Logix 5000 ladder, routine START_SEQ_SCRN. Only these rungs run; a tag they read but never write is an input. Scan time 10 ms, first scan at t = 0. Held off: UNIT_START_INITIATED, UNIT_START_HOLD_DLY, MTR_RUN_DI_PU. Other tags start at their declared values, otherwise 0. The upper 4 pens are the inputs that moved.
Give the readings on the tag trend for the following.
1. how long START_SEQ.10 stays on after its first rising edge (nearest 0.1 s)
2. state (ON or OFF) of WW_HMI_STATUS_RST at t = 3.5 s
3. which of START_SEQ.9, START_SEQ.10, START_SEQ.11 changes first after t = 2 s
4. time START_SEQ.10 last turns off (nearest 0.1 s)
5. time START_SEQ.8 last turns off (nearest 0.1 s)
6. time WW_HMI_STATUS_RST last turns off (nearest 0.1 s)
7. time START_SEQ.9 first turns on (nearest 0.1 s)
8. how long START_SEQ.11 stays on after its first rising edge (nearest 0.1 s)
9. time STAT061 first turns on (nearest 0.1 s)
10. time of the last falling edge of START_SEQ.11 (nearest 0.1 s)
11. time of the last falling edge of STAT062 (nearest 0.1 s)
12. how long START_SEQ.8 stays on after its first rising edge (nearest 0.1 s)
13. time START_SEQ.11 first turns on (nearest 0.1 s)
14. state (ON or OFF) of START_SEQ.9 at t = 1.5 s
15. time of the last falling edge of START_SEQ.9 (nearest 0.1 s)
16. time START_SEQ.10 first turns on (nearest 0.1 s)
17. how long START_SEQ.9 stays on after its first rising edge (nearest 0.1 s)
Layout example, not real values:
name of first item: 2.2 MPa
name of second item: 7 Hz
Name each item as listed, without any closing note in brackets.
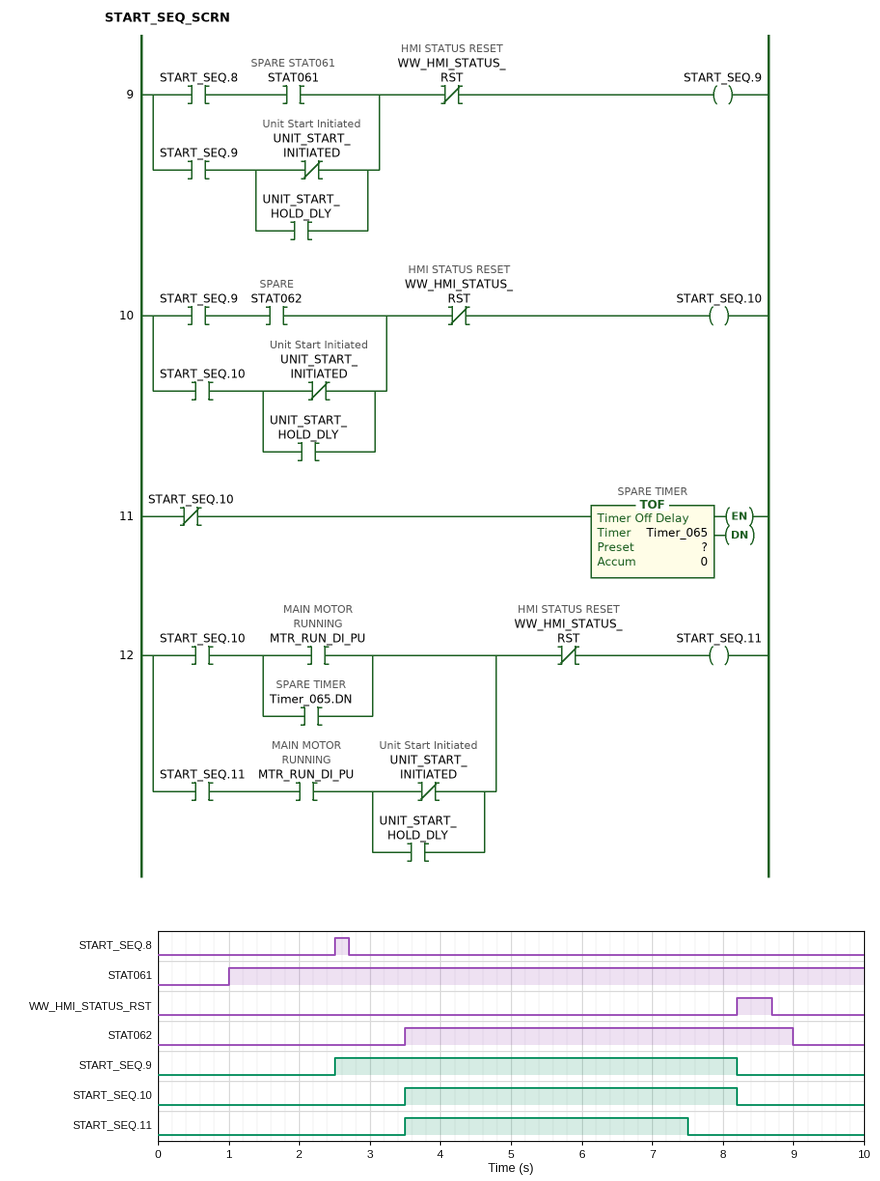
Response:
how long START_SEQ.10 stays on after its first rising edge: 4.7 s
state (ON or OFF) of WW_HMI_STATUS_RST at t = 3.5 s: OFF
which of START_SEQ.9, START_SEQ.10, START_SEQ.11 changes first after t = 2 s: START_SEQ.9
time START_SEQ.10 last turns off: 8.2 s
time START_SEQ.8 last turns off: 2.7 s
time WW_HMI_STATUS_RST last turns off: 8.7 s
time START_SEQ.9 first turns on: 2.5 s
how long START_SEQ.11 stays on after its first rising edge: 4.0 s
time STAT061 first turns on: 1.0 s
time of the last falling edge of START_SEQ.11: 7.5 s
time of the last falling edge of STAT062: 9.0 s
how long START_SEQ.8 stays on after its first rising edge: 0.2 s
time START_SEQ.11 first turns on: 3.5 s
state (ON or OFF) of START_SEQ.9 at t = 1.5 s: OFF
time of the last falling edge of START_SEQ.9: 8.2 s
time START_SEQ.10 first turns on: 3.5 s
how long START_SEQ.9 stays on after its first rising edge: 5.7 s
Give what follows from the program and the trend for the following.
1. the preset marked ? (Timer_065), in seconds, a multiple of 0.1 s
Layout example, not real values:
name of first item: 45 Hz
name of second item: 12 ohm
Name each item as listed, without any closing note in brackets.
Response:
the preset marked ? (Timer_065), in seconds, a multiple of 0.1 s: 4.0 s
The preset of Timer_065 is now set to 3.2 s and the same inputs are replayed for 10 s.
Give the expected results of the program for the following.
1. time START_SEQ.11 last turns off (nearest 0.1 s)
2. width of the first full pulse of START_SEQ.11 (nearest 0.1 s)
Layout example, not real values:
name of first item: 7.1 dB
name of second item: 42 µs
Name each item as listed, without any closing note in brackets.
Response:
time START_SEQ.11 last turns off: 6.7 s
width of the first full pulse of START_SEQ.11: 3.2 s
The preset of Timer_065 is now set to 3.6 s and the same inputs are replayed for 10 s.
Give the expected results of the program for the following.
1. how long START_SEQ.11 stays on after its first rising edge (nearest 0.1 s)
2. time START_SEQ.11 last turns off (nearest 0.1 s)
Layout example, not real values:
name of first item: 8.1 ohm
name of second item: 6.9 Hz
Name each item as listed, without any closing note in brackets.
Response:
how long START_SEQ.11 stays on after its first rising edge: 3.6 s
time START_SEQ.11 last turns off: 7.1 s
